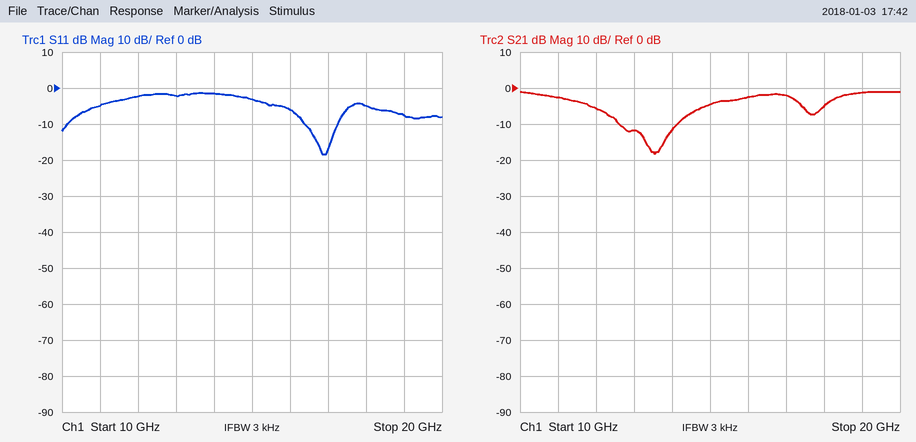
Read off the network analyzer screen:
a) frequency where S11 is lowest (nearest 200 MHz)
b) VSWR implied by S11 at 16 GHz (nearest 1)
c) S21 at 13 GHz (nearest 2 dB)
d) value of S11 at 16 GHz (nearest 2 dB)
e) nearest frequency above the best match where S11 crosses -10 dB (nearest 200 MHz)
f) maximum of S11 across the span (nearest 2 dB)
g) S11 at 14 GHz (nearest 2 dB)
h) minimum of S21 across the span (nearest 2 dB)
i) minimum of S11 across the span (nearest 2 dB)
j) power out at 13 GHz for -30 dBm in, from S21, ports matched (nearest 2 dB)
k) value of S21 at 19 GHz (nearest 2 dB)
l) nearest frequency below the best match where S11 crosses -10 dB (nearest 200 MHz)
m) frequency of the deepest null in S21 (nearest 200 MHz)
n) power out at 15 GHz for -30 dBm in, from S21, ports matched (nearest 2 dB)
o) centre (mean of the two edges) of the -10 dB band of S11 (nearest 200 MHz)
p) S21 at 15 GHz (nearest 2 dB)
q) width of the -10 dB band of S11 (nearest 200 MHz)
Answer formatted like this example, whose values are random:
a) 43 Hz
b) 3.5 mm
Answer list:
a) 16.8 GHz
b) 3
c) -12 dB
d) -6 dB
e) 17.2 GHz
f) -2 dB
g) -2 dB
h) -18 dB
i) -18 dB
j) -42 dBm
k) -2 dB
l) 16.4 GHz
m) 13.6 GHz
n) -34 dBm
o) 16.8 GHz
p) -4 dB
q) 800 MHz
